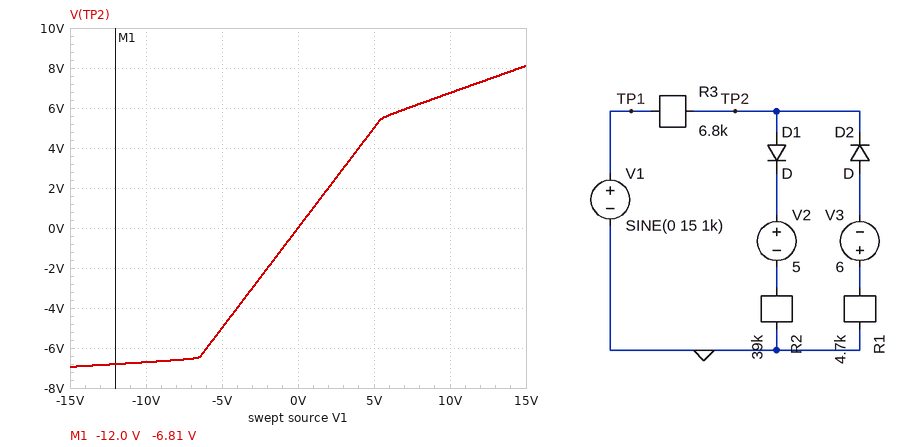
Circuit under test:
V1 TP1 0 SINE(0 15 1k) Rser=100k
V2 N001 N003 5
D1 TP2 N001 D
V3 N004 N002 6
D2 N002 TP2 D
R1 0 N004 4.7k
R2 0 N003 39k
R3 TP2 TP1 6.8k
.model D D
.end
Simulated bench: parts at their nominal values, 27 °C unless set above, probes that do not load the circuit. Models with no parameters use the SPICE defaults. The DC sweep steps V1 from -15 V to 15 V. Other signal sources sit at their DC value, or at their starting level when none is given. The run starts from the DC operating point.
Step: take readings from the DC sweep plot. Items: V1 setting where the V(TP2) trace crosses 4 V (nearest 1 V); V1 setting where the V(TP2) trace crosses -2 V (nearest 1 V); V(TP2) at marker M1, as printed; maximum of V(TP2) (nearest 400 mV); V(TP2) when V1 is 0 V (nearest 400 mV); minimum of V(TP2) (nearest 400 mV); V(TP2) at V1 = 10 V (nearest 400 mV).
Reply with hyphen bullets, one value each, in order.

- 4 V
- -2 V
- -6.81 V
- 8.0 V
- 0 V
- -6.8 V
- 6.8 V
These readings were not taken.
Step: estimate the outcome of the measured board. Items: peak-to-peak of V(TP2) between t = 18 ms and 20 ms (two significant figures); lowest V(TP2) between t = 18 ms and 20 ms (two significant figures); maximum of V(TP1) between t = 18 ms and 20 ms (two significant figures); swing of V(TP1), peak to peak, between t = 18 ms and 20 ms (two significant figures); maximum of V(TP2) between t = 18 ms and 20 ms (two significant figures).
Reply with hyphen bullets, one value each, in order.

- 15 V
- -6.9 V
- 8.5 V
- 16 V
- 8.1 V
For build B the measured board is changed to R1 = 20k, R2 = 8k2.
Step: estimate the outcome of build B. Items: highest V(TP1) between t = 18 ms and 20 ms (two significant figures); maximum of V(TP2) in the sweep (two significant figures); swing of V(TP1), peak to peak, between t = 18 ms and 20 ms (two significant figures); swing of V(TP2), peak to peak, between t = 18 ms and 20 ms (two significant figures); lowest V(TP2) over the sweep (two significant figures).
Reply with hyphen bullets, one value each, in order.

- 6.8 V
- 6.3 V
- 15 V
- 14 V
- -7.9 V
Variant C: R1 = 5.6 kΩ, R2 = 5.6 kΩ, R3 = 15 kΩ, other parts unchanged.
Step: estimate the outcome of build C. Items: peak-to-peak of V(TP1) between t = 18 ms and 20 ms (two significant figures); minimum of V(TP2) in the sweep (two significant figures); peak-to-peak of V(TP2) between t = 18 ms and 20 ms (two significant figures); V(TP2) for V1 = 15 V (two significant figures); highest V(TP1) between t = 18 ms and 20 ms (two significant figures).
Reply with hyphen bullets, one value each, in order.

- 15 V
- -7.0 V
- 13 V
- 6.0 V
- 7.2 V
